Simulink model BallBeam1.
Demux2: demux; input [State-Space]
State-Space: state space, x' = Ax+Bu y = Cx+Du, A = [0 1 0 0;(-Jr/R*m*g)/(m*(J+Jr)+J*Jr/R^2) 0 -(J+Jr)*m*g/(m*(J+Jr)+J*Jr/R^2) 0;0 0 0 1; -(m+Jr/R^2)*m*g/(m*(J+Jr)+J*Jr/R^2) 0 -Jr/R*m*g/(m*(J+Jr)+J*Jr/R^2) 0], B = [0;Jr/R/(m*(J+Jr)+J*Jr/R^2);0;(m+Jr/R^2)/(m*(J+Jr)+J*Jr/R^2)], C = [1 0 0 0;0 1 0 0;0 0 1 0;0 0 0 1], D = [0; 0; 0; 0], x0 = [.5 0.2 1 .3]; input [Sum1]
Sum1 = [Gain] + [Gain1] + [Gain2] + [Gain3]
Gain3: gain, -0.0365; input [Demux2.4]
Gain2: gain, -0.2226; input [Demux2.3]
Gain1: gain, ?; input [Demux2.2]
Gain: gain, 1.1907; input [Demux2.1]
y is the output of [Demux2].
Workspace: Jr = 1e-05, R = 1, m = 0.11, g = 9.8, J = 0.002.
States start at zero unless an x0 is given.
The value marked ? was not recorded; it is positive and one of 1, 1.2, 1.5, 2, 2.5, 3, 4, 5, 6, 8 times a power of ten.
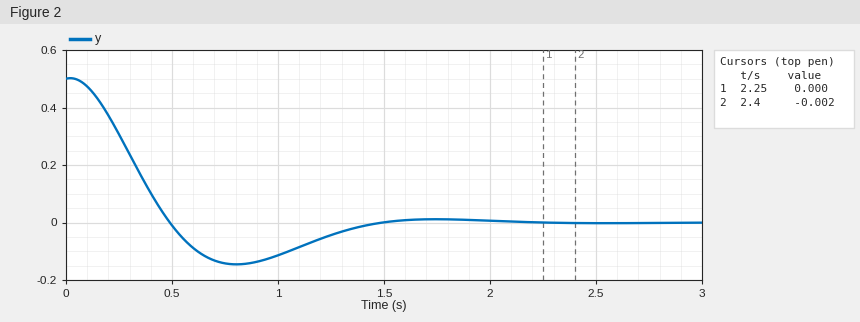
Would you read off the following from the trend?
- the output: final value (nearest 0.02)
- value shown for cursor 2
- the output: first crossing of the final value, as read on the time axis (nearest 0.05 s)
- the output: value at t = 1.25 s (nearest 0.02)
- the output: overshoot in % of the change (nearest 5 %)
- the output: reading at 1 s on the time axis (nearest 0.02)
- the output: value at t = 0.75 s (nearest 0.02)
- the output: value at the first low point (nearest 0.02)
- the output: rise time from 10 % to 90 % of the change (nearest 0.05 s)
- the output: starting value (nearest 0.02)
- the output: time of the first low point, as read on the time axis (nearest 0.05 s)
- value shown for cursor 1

0.00
-0.002
0.50 s
-0.04
30 %
-0.12
-0.14
-0.14
0.30 s
0.50
0.80 s
0.000
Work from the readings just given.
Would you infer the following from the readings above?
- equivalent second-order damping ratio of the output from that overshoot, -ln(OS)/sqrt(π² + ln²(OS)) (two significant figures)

0.36
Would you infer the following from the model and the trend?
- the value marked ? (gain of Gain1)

0.08
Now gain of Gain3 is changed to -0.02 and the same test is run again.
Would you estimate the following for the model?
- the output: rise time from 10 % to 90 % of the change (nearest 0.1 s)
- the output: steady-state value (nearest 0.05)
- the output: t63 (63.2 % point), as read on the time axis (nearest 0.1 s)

0.8 s
0.00
0.4 s
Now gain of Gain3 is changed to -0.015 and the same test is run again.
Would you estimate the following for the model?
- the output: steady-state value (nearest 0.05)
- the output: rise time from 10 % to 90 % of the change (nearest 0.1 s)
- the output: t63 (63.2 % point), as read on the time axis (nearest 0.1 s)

0.00
0.9 s
0.7 s
